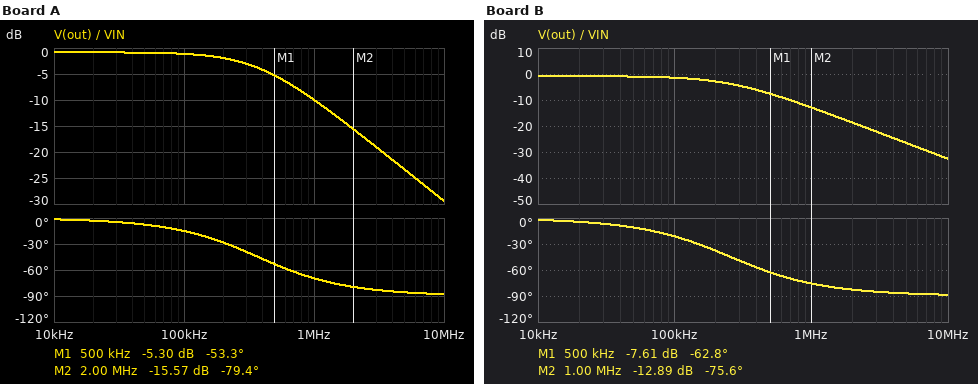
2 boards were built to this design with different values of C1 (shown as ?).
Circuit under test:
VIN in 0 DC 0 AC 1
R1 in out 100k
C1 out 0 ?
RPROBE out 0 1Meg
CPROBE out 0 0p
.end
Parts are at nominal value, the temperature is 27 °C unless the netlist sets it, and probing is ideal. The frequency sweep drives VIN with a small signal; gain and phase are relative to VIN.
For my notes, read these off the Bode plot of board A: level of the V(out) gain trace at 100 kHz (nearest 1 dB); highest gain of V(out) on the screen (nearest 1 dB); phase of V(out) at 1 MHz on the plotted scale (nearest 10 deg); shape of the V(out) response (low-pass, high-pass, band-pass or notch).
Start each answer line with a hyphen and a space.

- -1 dB
- -1 dB
- -70 deg
- low-pass
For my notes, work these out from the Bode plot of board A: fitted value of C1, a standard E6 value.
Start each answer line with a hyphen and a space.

- 4.7 pF
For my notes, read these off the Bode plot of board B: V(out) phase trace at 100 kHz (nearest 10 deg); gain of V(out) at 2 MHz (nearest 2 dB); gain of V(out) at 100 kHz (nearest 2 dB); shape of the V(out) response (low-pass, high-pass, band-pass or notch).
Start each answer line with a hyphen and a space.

- -20 deg
- -18 dB
- -2 dB
- low-pass
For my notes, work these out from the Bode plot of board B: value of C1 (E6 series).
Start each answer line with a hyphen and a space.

- 6.8 pF
